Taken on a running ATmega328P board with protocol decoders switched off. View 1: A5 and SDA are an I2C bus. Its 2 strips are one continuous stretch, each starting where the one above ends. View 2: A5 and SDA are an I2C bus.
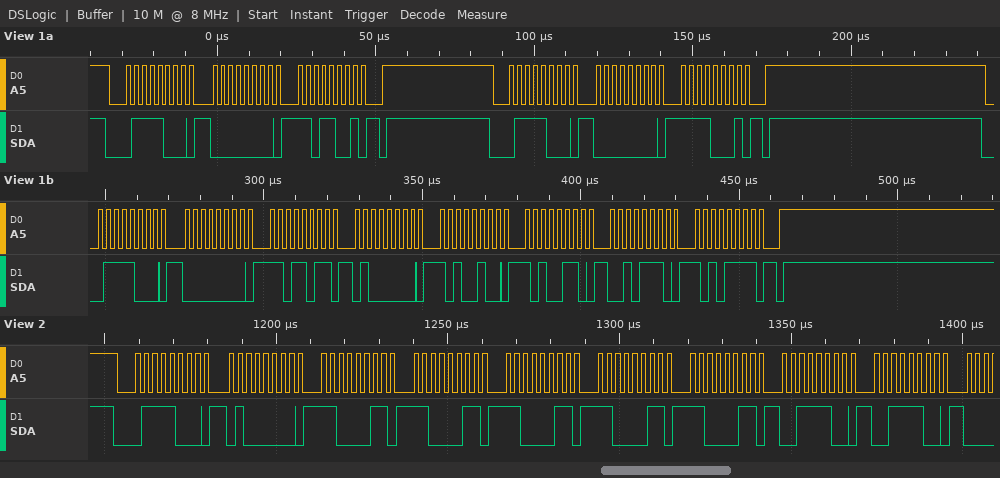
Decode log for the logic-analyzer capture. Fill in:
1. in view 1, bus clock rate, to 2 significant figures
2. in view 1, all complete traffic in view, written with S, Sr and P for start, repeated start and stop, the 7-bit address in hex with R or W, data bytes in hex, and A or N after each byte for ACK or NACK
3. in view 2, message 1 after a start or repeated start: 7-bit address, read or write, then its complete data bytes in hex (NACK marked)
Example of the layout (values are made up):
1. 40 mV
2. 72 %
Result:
1. 400 kHz
2. S 3CW A 00 A D9 A P S 3CW A 00 A F1 A P S 3CW A 00 A DB A 40 A A4 A A6 A 2E A AF A P
3. 0x3C write: 40 C3 C3 C3 C3 C3 3C 3C
